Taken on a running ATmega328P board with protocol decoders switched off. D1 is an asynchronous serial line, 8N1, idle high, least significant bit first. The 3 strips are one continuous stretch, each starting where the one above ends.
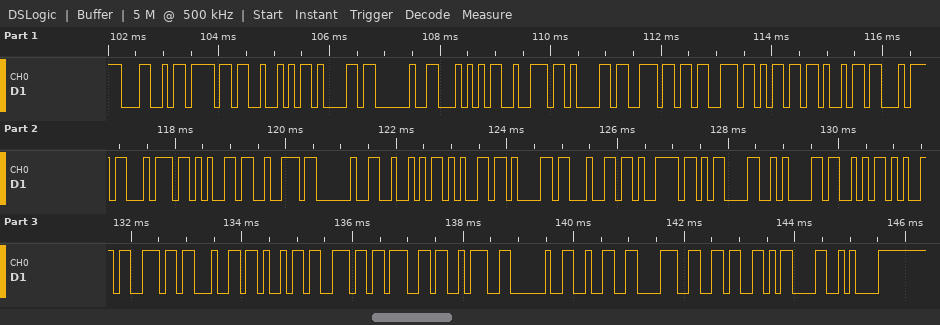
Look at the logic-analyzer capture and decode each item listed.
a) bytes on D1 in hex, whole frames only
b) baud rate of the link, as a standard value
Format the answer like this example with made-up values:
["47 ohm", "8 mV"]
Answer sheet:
["0x4C 0x6F 0x52 0x61 0x20 0x54 0x72 0x61 0x6E 0x73 0x6D 0x69 0x74 0x74 0x65 0x72 0x20 0x52 0x65 0x61 0x64 0x79 0x0D 0x0A 0x53 0x65 0x6E 0x64 0x69 0x6E 0x67 0x3A 0x20 0x32 0x38 0x36 0x0D 0x0A", "9600 baud"]
